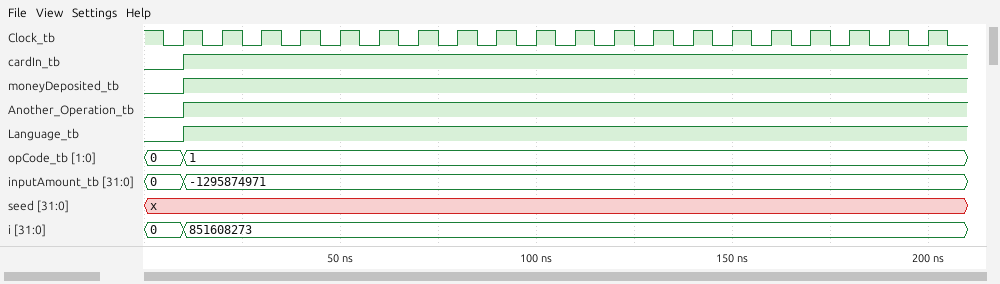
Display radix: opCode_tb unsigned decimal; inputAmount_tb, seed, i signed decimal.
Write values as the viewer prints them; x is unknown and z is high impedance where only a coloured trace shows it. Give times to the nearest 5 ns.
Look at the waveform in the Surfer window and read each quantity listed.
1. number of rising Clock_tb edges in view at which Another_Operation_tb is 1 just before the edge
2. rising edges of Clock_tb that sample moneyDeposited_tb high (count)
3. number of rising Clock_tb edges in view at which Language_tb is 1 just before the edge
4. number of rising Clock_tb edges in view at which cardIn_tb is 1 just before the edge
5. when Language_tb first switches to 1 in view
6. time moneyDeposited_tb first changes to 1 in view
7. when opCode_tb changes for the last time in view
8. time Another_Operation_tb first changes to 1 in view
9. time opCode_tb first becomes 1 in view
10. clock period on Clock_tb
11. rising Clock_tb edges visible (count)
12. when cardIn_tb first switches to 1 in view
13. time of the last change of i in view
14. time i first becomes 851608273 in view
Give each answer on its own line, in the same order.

19
19
19
19
10 ns
10 ns
10 ns
10 ns
10 ns
10 ns
20
10 ns
10 ns
10 ns
